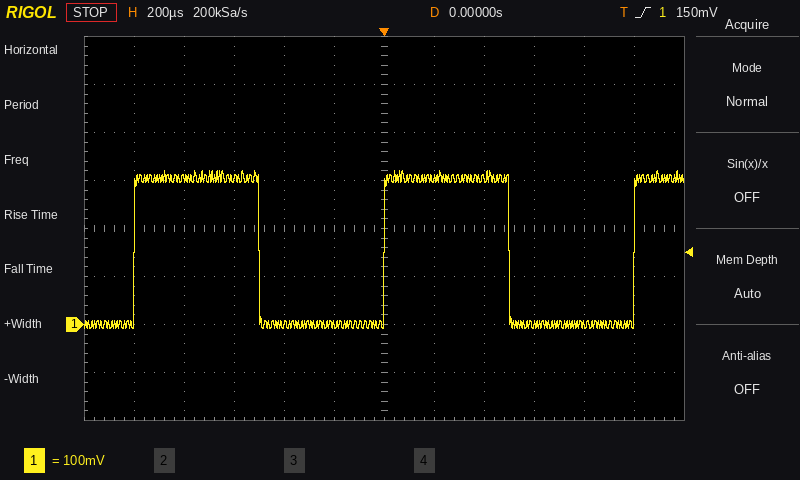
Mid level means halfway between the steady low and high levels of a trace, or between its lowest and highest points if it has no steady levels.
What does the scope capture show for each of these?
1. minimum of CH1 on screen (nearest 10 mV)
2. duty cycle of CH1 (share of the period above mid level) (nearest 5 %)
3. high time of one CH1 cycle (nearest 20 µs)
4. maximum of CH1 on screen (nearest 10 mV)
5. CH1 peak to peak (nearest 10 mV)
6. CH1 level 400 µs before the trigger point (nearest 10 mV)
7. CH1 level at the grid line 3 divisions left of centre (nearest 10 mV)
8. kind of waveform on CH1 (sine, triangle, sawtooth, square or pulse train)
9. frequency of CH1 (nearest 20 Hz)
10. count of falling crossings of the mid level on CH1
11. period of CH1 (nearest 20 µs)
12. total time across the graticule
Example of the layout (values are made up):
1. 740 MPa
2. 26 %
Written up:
1. -10 mV
2. 50 %
3. 500 µs
4. 320 mV
5. 330 mV
6. 0 mV
7. 300 mV
8. square
9. 1.00 kHz
10. 2
11. 1.00 ms
12. 2.4 ms
